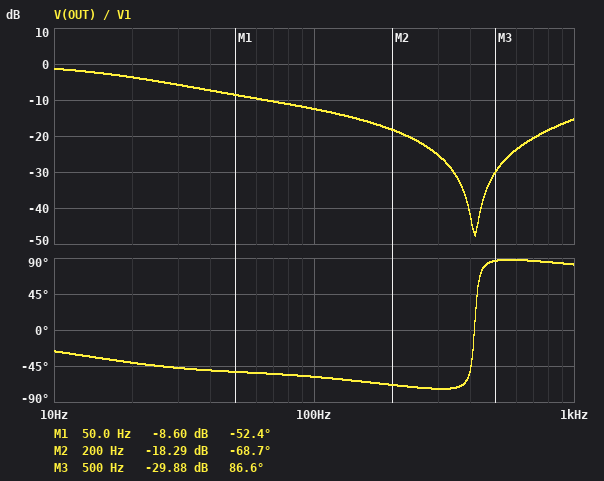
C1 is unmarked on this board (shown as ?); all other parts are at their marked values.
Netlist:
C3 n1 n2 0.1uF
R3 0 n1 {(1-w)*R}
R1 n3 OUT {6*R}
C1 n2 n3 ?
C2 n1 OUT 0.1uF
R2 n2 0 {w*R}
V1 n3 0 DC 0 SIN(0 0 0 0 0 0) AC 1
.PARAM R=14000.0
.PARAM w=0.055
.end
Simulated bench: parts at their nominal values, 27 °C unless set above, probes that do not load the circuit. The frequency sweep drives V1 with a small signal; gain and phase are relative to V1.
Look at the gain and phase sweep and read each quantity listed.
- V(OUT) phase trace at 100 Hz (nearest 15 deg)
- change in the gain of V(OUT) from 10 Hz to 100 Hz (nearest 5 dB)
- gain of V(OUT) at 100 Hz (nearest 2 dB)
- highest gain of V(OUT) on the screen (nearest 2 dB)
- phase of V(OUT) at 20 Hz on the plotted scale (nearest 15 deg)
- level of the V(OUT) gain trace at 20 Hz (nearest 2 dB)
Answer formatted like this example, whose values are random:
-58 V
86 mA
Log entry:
-60 deg
-10 dB
-12 dB
-2 dB
-45 deg
-4 dB
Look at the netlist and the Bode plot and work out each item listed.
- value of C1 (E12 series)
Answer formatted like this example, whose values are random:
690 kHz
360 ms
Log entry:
47 nF
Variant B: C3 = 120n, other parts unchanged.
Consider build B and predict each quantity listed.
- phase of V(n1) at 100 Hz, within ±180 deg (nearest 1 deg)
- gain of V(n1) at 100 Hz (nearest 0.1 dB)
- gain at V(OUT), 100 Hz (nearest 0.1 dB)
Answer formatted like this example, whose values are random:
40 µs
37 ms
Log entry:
-27 deg
-21.5 dB
-12.6 dB
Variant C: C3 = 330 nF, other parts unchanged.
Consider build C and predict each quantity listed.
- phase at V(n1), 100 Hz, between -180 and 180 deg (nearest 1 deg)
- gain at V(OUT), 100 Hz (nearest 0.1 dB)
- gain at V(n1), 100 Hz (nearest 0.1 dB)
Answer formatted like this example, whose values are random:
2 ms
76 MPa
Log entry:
-36 deg
-13.7 dB
-29.9 dB
